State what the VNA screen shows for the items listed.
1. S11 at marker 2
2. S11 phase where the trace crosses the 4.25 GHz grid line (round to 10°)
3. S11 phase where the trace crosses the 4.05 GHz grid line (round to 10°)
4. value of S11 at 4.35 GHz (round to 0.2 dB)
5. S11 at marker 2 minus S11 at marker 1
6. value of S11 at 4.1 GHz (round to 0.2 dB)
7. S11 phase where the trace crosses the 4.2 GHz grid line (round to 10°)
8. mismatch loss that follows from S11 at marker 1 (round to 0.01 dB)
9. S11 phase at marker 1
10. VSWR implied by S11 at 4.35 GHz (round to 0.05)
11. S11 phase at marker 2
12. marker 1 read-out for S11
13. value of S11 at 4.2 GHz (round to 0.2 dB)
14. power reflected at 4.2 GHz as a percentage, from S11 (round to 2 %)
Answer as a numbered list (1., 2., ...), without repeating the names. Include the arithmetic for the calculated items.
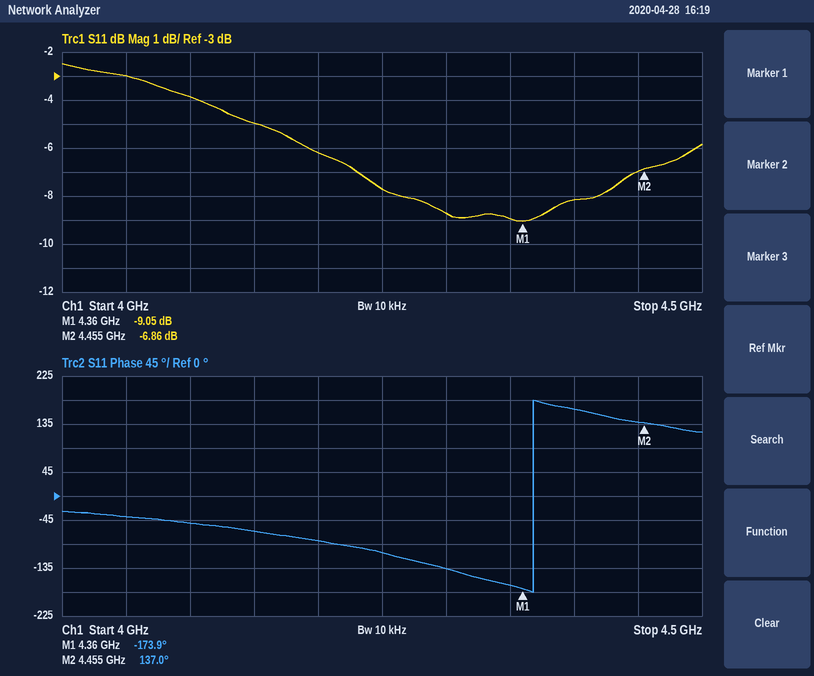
1. -6.86 dB
2. -110°
3. -40°
4. -9.0 dB
5. -6.86 − (-9.05) = 2.19 dB
6. -3.8 dB
7. -80°
8. −10 log10(1 − 10^(-9.05/10)) ≈ 0.58 dB
9. -173.9°
10. |Γ| = 10^(-9/20) = 0.3548; VSWR = (1 + 0.3548)/(1 − 0.3548) ≈ 2.10
11. 137.0°
12. -9.05 dB
13. -6.2 dB
14. 10^(-6.2/10) ≈ 24 %
